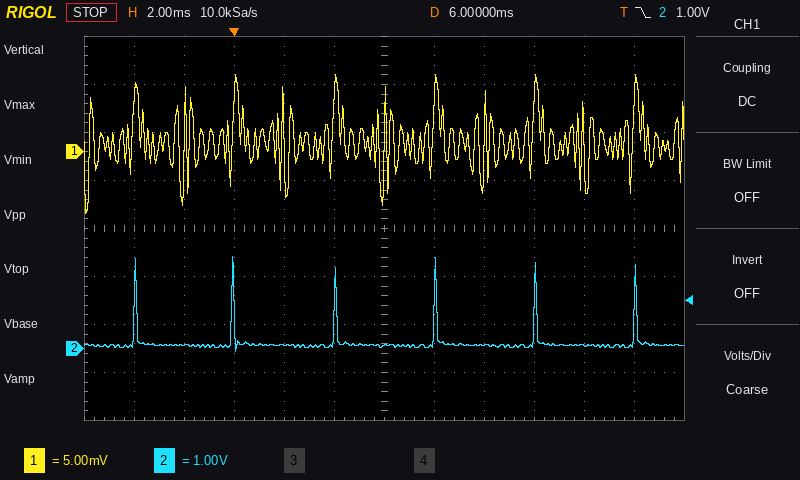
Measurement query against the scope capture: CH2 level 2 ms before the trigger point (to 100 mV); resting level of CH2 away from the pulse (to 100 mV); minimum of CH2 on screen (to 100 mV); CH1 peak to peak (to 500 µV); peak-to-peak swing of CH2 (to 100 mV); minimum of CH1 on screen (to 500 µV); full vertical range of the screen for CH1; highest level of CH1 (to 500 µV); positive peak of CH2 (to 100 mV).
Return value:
100 mV
100 mV
-100 mV
14.5 mV
2.0 V
-6.5 mV
40 mV
8.0 mV
1.9 V
